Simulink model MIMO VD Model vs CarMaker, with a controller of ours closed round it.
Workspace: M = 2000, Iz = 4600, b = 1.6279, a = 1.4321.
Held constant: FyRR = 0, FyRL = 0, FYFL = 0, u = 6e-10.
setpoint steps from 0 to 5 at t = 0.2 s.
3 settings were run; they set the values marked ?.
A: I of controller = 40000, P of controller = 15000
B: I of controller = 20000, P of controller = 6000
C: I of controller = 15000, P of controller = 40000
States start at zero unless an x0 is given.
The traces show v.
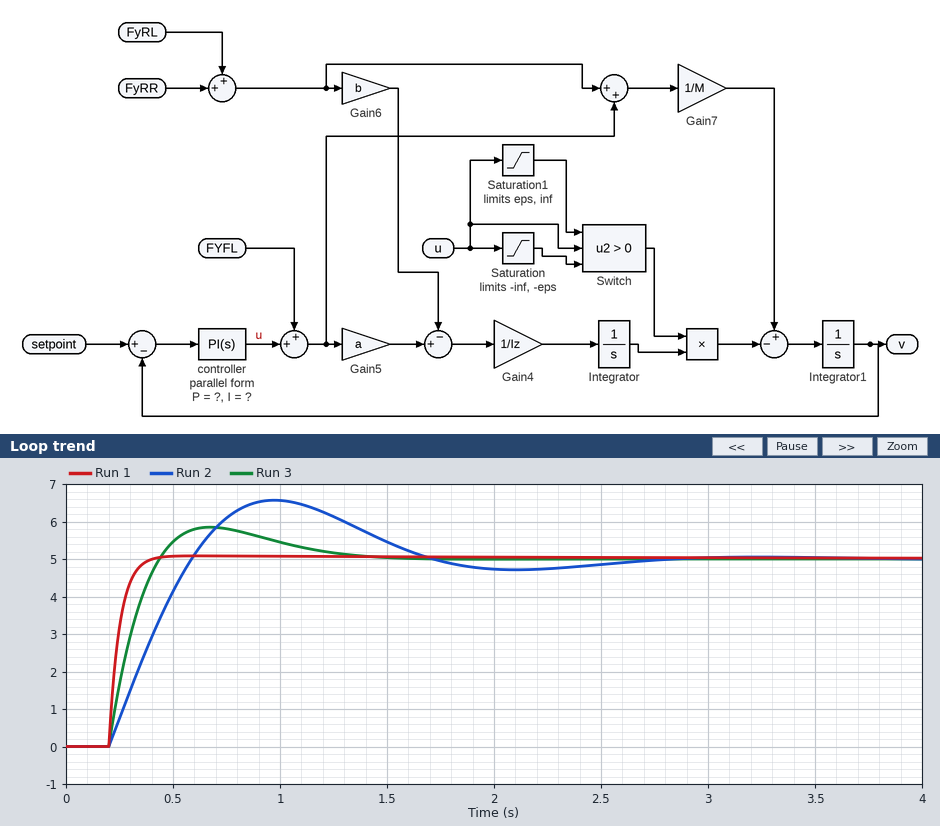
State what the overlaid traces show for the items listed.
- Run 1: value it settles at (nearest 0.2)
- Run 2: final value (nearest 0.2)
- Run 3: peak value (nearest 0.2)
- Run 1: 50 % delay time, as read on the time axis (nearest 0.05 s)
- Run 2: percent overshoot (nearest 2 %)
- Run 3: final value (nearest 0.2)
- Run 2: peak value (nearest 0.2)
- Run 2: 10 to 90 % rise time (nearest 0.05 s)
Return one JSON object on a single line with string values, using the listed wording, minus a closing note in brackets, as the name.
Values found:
{"Run 1: value it settles at": "5.0", "Run 2: final value": "5.0", "Run 3: peak value": "5.8", "Run 1: 50 % delay time, as read on the time axis": "0.25 s", "Run 2: percent overshoot": "32 %", "Run 3: final value": "5.0", "Run 2: peak value": "6.6", "Run 2: 10 to 90 % rise time": "0.30 s"}
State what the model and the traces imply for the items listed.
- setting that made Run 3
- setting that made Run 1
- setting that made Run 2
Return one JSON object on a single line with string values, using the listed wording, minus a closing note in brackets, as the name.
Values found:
{"setting that made Run 3": "A", "setting that made Run 1": "C", "setting that made Run 2": "B"}
